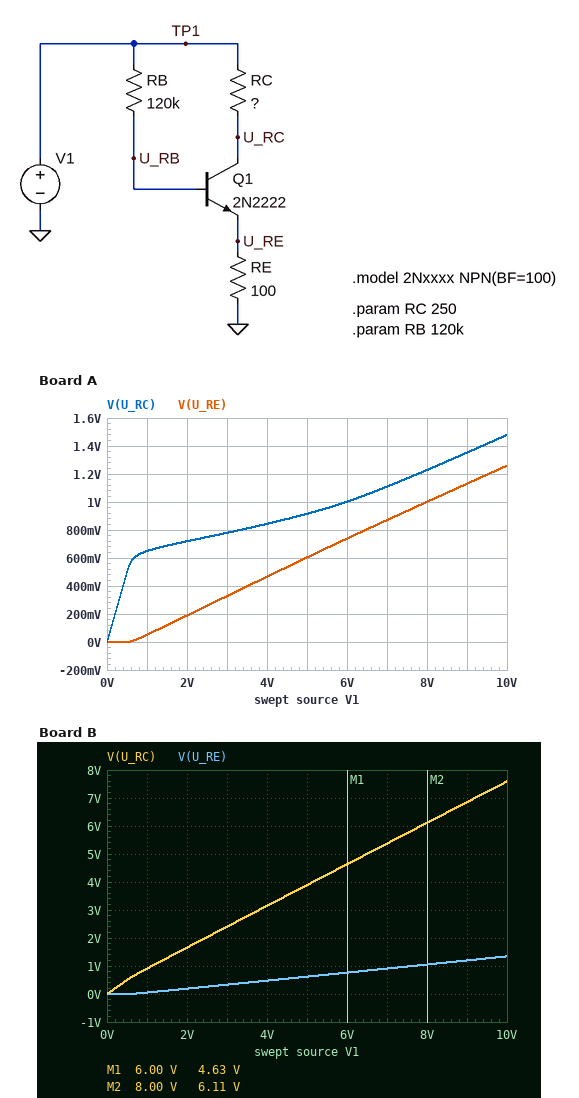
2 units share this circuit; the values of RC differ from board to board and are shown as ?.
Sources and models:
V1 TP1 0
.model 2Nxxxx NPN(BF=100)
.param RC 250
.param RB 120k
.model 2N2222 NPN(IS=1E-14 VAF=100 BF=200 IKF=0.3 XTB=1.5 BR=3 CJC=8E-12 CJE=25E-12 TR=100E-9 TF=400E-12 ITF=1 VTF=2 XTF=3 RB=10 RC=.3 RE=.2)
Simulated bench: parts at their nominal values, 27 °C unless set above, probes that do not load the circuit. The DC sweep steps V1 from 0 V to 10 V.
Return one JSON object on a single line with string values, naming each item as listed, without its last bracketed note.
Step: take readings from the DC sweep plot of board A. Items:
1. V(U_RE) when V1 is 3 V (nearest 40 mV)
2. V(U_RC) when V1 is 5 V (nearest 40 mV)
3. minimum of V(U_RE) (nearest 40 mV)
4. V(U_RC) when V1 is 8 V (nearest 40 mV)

{"V(U_RE) when V1 is 3 V": "320 mV", "V(U_RC) when V1 is 5 V": "920 mV", "minimum of V(U_RE)": "0 V", "V(U_RC) when V1 is 8 V": "1.24 V"}
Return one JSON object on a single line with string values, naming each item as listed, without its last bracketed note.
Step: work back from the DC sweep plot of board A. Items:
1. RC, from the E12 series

{"RC, from the E12 series": "680 Ω"}
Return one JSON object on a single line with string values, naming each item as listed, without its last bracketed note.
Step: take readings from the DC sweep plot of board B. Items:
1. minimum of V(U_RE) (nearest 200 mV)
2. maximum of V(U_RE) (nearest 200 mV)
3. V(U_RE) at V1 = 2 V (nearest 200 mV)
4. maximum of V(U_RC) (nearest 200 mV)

{"minimum of V(U_RE)": "0 V", "maximum of V(U_RE)": "1.4 V", "V(U_RE) at V1 = 2 V": "200 mV", "maximum of V(U_RC)": "7.6 V"}
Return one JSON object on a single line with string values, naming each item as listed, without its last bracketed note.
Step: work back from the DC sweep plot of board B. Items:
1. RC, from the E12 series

{"RC, from the E12 series": "180 Ω"}
